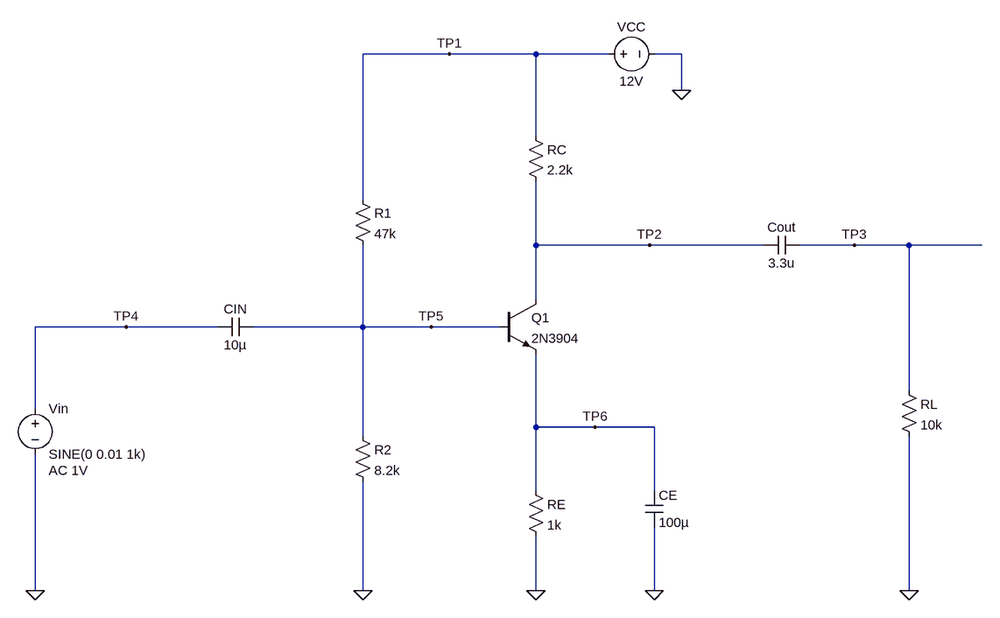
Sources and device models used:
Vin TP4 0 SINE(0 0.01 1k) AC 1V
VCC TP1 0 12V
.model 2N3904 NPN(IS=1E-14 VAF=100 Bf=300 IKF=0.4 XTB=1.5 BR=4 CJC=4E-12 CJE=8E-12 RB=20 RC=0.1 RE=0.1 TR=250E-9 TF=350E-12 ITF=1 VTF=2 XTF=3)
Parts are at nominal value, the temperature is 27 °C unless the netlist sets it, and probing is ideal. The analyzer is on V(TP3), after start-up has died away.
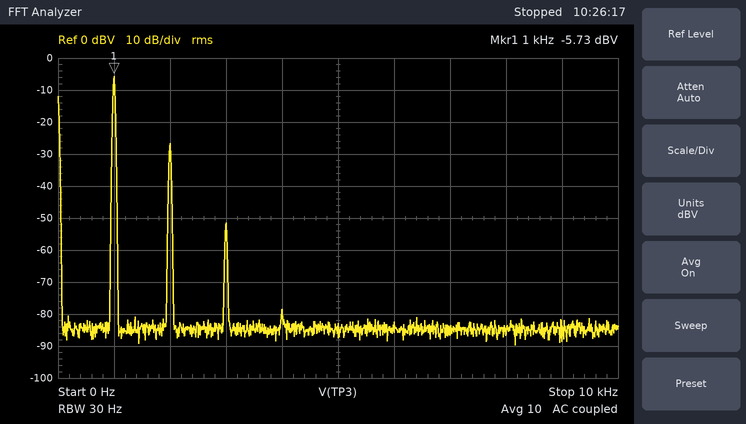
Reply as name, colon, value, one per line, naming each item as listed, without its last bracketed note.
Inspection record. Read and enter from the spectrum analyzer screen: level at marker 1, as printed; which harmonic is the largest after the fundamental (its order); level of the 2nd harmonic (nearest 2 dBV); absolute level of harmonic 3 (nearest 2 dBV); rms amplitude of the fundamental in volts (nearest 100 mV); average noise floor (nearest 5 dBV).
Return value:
level at marker 1, as printed: -5.73 dBV
which harmonic is the largest after the fundamental: 2
level of the 2nd harmonic: -26 dBV
absolute level of harmonic 3: -52 dBV
rms amplitude of the fundamental in volts: 500 mV
average noise floor: -85 dBV
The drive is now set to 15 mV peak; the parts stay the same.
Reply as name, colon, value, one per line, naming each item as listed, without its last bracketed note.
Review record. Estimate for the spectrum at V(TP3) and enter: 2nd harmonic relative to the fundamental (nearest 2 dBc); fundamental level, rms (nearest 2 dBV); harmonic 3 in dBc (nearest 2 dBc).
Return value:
2nd harmonic relative to the fundamental: -18 dBc
fundamental level, rms: -2 dBV
harmonic 3 in dBc: -38 dBc
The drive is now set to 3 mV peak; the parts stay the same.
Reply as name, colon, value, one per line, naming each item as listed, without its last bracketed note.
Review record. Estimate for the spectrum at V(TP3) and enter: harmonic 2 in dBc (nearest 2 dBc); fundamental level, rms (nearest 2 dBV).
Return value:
harmonic 2 in dBc: -32 dBc
fundamental level, rms: -16 dBV
